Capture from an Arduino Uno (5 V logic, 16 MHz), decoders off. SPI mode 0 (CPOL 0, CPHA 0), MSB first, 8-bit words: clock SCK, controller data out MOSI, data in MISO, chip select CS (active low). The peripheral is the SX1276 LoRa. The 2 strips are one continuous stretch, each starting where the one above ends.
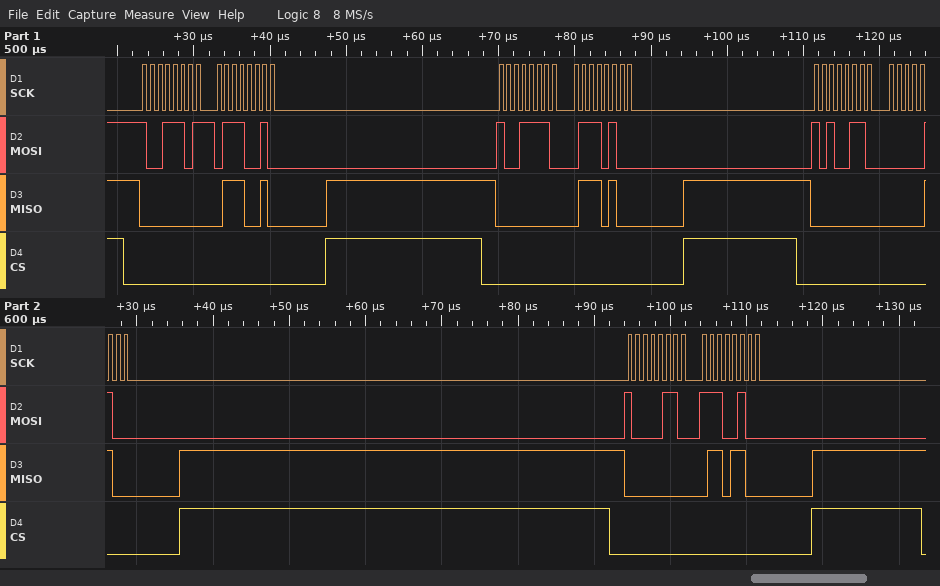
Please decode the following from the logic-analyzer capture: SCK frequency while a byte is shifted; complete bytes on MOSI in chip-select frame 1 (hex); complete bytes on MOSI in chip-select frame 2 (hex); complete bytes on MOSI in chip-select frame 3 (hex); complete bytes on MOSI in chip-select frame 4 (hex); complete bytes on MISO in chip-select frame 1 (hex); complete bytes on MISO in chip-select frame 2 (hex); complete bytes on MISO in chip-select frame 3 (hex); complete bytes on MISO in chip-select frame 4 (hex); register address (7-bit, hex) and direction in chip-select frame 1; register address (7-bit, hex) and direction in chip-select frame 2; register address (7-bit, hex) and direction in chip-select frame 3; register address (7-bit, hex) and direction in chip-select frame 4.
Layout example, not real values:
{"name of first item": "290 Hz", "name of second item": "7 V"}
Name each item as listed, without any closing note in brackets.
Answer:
{"SCK frequency while a byte is shifted": "1 MHz", "complete bytes on MOSI in chip-select frame 1": "9D 72", "complete bytes on MOSI in chip-select frame 2": "9E 74", "complete bytes on MOSI in chip-select frame 3": "A6 04", "complete bytes on MOSI in chip-select frame 4": "86 E4", "complete bytes on MISO in chip-select frame 1": "00 72", "complete bytes on MISO in chip-select frame 2": "00 74", "complete bytes on MISO in chip-select frame 3": "00 04", "complete bytes on MISO in chip-select frame 4": "00 6C", "register address (7-bit, hex) and direction in chip-select frame 1": "0x1D write", "register address (7-bit, hex) and direction in chip-select frame 2": "0x1E write", "register address (7-bit, hex) and direction in chip-select frame 3": "0x26 write", "register address (7-bit, hex) and direction in chip-select frame 4": "0x06 write"}
